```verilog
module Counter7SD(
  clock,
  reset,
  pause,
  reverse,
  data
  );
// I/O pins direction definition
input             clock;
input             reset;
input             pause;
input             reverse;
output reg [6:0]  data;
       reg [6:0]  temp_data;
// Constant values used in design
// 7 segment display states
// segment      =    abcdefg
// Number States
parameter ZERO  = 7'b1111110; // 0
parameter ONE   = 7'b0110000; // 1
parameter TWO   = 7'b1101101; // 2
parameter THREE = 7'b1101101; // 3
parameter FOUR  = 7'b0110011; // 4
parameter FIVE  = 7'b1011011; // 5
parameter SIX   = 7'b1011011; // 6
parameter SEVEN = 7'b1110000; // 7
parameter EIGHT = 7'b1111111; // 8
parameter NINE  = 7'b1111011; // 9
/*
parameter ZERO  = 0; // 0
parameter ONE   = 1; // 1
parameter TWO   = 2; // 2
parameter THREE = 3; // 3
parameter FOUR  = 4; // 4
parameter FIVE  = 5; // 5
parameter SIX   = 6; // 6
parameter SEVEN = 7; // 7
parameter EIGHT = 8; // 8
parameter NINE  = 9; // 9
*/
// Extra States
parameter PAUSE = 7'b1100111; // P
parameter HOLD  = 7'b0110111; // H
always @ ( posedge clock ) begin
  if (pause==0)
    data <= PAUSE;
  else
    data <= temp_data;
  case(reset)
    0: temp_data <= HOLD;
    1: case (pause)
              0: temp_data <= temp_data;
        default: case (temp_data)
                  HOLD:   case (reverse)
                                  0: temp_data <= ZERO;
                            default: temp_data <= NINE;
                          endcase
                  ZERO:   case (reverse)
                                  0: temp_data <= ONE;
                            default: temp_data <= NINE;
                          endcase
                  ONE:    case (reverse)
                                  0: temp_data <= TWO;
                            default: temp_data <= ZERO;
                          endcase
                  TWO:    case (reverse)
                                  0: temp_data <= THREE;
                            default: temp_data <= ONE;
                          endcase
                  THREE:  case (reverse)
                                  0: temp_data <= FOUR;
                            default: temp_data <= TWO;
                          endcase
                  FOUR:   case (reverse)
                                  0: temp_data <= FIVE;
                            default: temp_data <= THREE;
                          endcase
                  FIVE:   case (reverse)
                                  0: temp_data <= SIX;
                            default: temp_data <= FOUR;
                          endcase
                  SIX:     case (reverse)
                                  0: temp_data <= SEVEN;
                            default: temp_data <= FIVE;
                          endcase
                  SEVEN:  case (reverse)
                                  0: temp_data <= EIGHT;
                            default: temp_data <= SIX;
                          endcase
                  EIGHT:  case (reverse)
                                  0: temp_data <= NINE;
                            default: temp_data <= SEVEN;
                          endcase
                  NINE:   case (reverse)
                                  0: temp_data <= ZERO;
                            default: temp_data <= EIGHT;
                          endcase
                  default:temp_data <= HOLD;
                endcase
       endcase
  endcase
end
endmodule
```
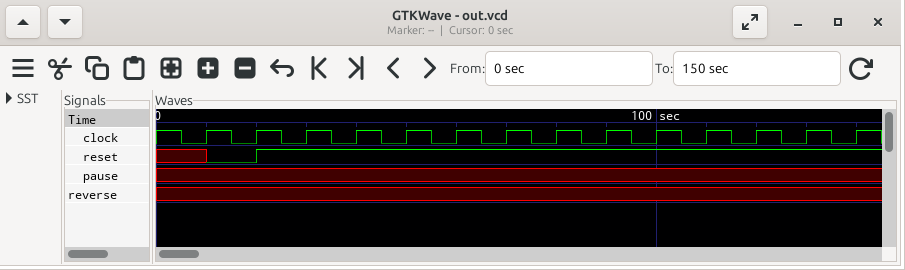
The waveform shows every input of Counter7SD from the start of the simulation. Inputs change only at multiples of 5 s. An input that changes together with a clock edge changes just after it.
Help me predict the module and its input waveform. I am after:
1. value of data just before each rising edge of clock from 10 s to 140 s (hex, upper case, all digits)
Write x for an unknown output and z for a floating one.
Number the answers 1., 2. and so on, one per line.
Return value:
1. x, x, x, 37, 7B, 7F, 70, 5B, 33, 6D, 30, 7E, 7B, 7F
